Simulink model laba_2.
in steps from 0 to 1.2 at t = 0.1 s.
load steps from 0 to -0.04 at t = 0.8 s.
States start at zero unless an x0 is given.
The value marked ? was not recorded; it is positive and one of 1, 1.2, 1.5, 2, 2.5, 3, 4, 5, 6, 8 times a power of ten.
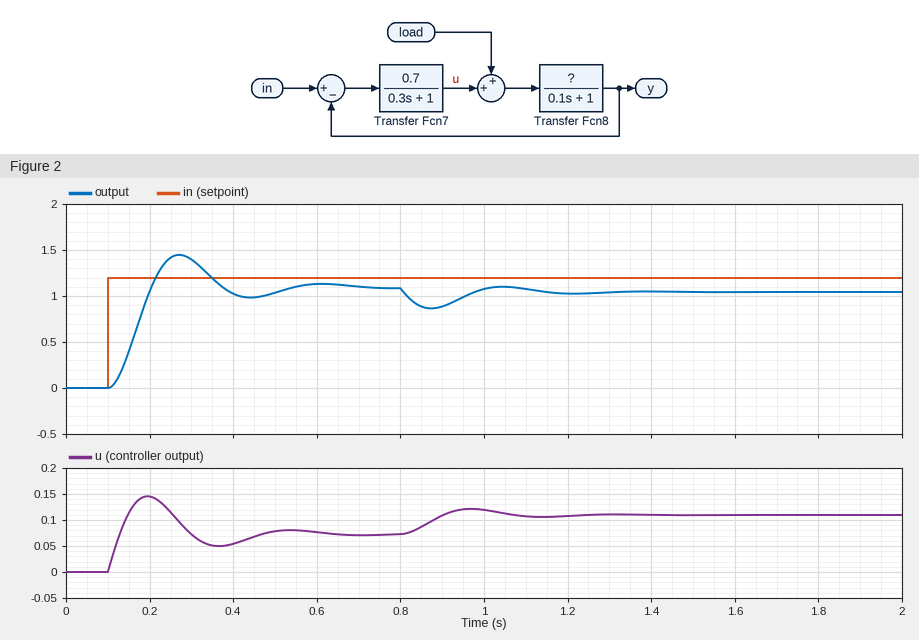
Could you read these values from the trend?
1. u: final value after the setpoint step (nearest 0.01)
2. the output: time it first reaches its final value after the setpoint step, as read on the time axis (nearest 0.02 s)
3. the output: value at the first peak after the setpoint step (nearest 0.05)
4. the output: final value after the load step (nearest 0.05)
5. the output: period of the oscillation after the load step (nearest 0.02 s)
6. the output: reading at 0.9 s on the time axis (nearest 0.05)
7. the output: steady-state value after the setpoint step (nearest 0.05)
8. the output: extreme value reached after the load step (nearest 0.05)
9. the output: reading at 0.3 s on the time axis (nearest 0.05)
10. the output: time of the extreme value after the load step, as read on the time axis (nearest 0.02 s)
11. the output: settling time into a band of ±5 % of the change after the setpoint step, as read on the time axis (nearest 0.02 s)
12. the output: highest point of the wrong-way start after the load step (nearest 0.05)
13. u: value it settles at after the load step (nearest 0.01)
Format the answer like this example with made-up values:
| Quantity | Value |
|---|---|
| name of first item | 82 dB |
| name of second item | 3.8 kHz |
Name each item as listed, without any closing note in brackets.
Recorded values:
| Quantity | Value |
|---|---|
| u: final value after the setpoint step | 0.07 |
| the output: time it first reaches its final value after the setpoint step, as read on the time axis | 0.20 s |
| the output: value at the first peak after the setpoint step | 1.45 |
| the output: final value after the load step | 1.05 |
| the output: period of the oscillation after the load step | 0.34 s |
| the output: reading at 0.9 s on the time axis | 0.90 |
| the output: steady-state value after the setpoint step | 1.10 |
| the output: extreme value reached after the load step | 0.85 |
| the output: reading at 0.3 s on the time axis | 1.40 |
| the output: time of the extreme value after the load step, as read on the time axis | 0.88 s |
| the output: settling time into a band of ±5 % of the change after the setpoint step, as read on the time axis | 0.50 s |
| the output: highest point of the wrong-way start after the load step | 1.10 |
| u: value it settles at after the load step | 0.11 |
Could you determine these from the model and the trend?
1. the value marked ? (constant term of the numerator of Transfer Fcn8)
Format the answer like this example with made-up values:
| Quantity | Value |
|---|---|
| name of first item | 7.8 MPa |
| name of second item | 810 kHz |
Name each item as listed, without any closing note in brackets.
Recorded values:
| Quantity | Value |
|---|---|
| the value marked ? | 15 |
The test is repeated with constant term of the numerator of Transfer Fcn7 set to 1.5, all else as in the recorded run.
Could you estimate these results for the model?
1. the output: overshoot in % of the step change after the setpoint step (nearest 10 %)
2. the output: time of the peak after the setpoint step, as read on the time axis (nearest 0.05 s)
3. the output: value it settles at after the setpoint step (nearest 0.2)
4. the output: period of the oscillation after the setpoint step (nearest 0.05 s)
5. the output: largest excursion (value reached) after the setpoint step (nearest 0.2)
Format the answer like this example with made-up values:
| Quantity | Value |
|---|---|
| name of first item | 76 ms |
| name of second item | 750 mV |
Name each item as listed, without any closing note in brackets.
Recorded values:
| Quantity | Value |
|---|---|
| the output: overshoot in % of the step change after the setpoint step | 50 % |
| the output: time of the peak after the setpoint step, as read on the time axis | 0.20 s |
| the output: value it settles at after the setpoint step | 1.2 |
| the output: period of the oscillation after the setpoint step | 0.25 s |
| the output: largest excursion (value reached) after the setpoint step | 1.6 |
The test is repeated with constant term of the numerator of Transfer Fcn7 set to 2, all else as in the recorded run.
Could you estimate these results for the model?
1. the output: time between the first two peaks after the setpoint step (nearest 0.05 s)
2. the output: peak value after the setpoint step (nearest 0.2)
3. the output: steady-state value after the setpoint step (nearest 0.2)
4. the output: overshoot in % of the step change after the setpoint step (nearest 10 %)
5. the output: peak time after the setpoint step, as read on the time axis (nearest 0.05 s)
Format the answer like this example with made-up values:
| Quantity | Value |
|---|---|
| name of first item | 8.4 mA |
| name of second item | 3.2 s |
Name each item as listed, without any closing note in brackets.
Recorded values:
| Quantity | Value |
|---|---|
| the output: time between the first two peaks after the setpoint step | 0.20 s |
| the output: peak value after the setpoint step | 1.8 |
| the output: steady-state value after the setpoint step | 1.2 |
| the output: overshoot in % of the step change after the setpoint step | 50 % |
| the output: peak time after the setpoint step, as read on the time axis | 0.20 s |
